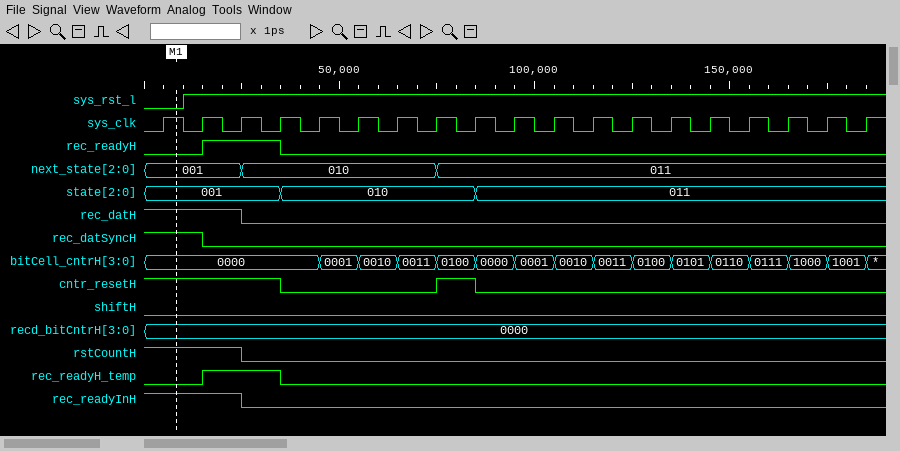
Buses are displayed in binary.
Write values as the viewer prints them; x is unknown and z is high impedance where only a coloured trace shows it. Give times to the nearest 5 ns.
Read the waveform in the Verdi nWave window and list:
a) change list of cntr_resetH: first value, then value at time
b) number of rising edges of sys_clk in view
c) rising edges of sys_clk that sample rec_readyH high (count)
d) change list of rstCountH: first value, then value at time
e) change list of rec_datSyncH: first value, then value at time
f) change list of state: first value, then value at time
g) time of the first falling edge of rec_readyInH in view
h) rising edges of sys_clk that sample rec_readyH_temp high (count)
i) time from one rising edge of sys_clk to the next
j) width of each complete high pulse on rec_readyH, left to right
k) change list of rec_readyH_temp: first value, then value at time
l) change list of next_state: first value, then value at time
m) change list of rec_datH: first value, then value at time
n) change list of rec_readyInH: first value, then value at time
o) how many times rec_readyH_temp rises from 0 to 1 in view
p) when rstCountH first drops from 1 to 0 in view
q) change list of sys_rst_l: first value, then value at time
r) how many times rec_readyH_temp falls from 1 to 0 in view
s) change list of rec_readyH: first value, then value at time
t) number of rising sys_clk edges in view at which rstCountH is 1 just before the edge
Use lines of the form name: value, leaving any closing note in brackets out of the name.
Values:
change list of cntr_resetH: first value, then value at time: 1, 0 at 35 ns, 1 at 75 ns, 0 at 85 ns
number of rising edges of sys_clk in view: 19
rising edges of sys_clk that sample rec_readyH high: 2
change list of rstCountH: first value, then value at time: 1, 0 at 25 ns
change list of rec_datSyncH: first value, then value at time: 1, 0 at 15 ns
change list of state: first value, then value at time: 001, 010 at 35 ns, 011 at 85 ns
time of the first falling edge of rec_readyInH in view: 25 ns
rising edges of sys_clk that sample rec_readyH_temp high: 2
time from one rising edge of sys_clk to the next: 10 ns
width of each complete high pulse on rec_readyH, left to right: 20 ns
change list of rec_readyH_temp: first value, then value at time: 0, 1 at 15 ns, 0 at 35 ns
change list of next_state: first value, then value at time: 001, 010 at 25 ns, 011 at 75 ns
change list of rec_datH: first value, then value at time: 1, 0 at 25 ns
change list of rec_readyInH: first value, then value at time: 1, 0 at 25 ns
how many times rec_readyH_temp rises from 0 to 1 in view: 1
when rstCountH first drops from 1 to 0 in view: 25 ns
change list of sys_rst_l: first value, then value at time: 0, 1 at 10 ns
how many times rec_readyH_temp falls from 1 to 0 in view: 1
change list of rec_readyH: first value, then value at time: 0, 1 at 15 ns, 0 at 35 ns
number of rising sys_clk edges in view at which rstCountH is 1 just before the edge: 3
